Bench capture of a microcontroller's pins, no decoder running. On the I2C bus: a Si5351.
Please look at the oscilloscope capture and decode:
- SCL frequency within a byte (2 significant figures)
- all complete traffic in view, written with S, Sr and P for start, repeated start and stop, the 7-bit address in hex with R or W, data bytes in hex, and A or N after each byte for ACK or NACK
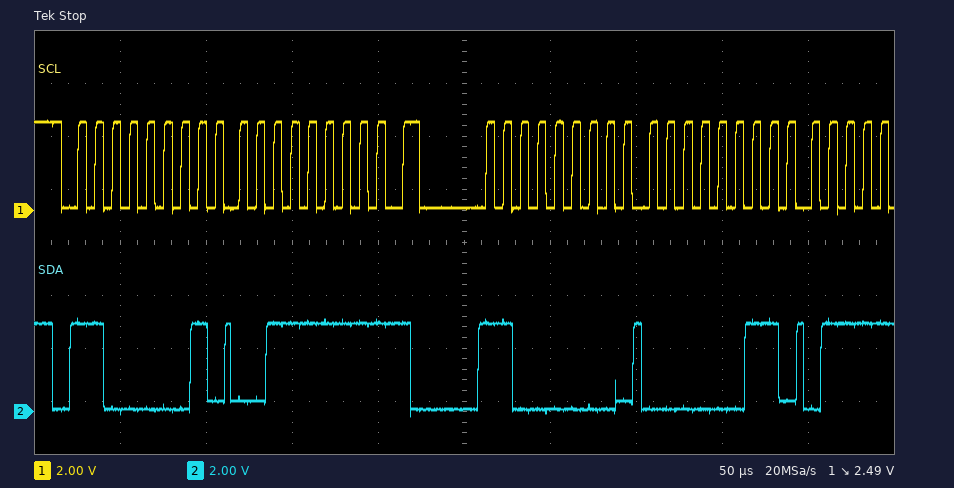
100 kHz
S 60R A 3F N Sr 60W A 03 A
